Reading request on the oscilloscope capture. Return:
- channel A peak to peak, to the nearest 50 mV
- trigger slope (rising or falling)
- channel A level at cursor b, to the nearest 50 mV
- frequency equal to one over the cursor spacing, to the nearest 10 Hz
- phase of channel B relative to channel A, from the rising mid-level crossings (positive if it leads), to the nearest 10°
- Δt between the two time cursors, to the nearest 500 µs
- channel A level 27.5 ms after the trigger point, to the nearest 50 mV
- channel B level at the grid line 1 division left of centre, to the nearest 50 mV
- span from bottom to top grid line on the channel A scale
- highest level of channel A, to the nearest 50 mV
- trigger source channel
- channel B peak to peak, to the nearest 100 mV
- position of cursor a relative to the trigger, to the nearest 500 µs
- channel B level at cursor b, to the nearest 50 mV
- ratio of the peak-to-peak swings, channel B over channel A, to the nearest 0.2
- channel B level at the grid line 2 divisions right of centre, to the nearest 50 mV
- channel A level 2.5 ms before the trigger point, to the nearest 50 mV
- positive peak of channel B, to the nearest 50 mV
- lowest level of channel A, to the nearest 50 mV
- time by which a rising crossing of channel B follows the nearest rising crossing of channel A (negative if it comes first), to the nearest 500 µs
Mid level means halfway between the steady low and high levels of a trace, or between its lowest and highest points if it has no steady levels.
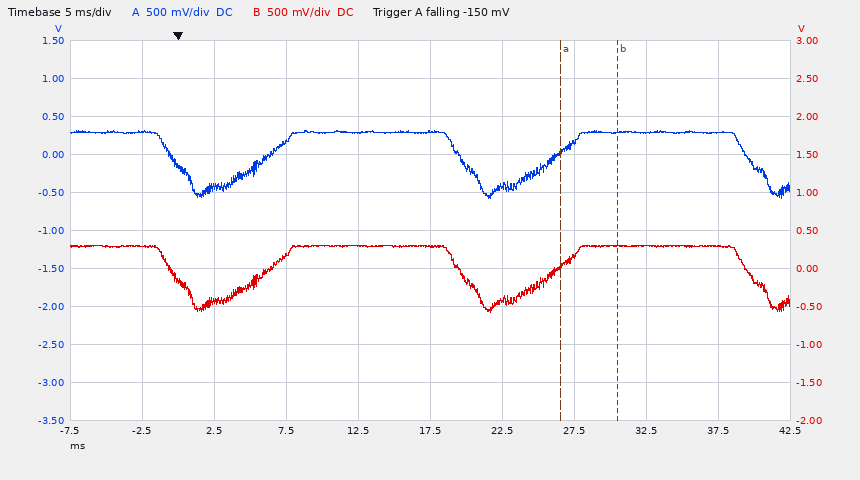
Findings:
900 mV
falling
300 mV
250 Hz
0°
4.0 ms
150 mV
300 mV
5 V
300 mV
channel A
900 mV
+26.5 ms
300 mV
1.0
150 mV
300 mV
300 mV
-600 mV
0.0 ms
